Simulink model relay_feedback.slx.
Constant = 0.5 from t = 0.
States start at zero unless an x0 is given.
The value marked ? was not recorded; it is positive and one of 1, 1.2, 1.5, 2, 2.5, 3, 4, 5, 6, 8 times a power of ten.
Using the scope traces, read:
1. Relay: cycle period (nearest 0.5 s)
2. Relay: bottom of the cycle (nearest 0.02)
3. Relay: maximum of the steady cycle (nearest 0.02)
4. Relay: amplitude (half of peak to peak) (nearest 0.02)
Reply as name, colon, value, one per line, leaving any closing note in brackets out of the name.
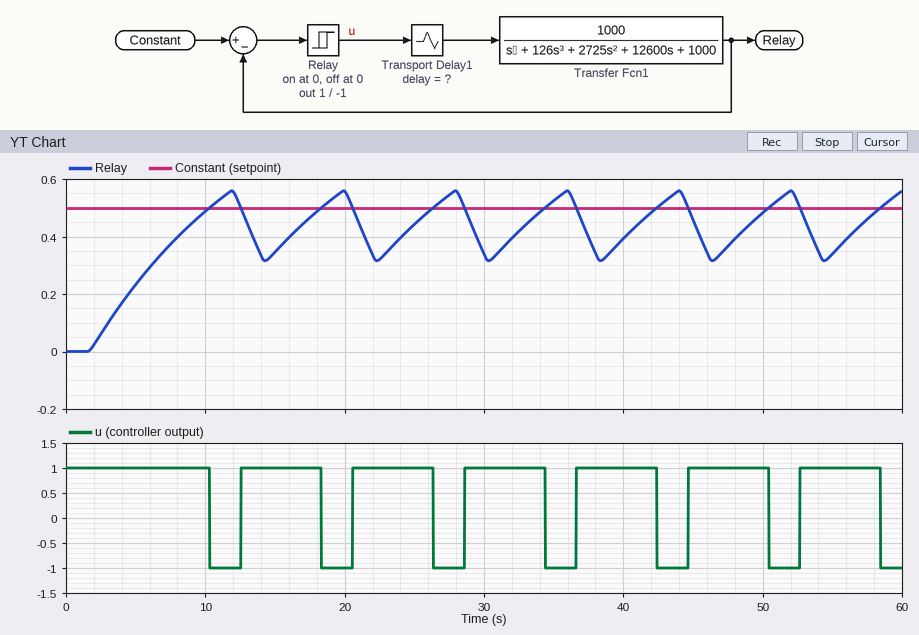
Relay: cycle period: 8.0 s
Relay: bottom of the cycle: 0.32
Relay: maximum of the steady cycle: 0.56
Relay: amplitude (half of peak to peak): 0.12
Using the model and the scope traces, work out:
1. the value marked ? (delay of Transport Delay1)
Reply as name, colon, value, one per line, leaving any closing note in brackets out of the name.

the value marked ?: 1.5
